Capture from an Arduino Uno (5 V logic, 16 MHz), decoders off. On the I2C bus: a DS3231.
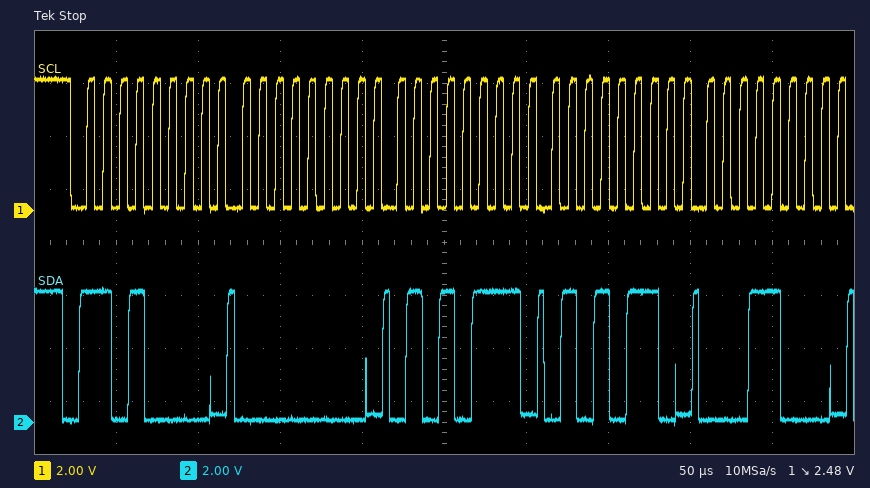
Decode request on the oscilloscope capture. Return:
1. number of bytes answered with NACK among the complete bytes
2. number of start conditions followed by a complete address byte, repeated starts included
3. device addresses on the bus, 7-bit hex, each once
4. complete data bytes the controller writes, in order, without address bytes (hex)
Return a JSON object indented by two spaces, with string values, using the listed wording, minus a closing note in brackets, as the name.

{
  "number of bytes answered with NACK among the complete bytes": "0",
  "number of start conditions followed by a complete address byte, repeated starts included": "1",
  "device addresses on the bus, 7-bit hex, each once": "0x68",
  "complete data bytes the controller writes, in order, without address bytes": "00 57 56 18"
}
